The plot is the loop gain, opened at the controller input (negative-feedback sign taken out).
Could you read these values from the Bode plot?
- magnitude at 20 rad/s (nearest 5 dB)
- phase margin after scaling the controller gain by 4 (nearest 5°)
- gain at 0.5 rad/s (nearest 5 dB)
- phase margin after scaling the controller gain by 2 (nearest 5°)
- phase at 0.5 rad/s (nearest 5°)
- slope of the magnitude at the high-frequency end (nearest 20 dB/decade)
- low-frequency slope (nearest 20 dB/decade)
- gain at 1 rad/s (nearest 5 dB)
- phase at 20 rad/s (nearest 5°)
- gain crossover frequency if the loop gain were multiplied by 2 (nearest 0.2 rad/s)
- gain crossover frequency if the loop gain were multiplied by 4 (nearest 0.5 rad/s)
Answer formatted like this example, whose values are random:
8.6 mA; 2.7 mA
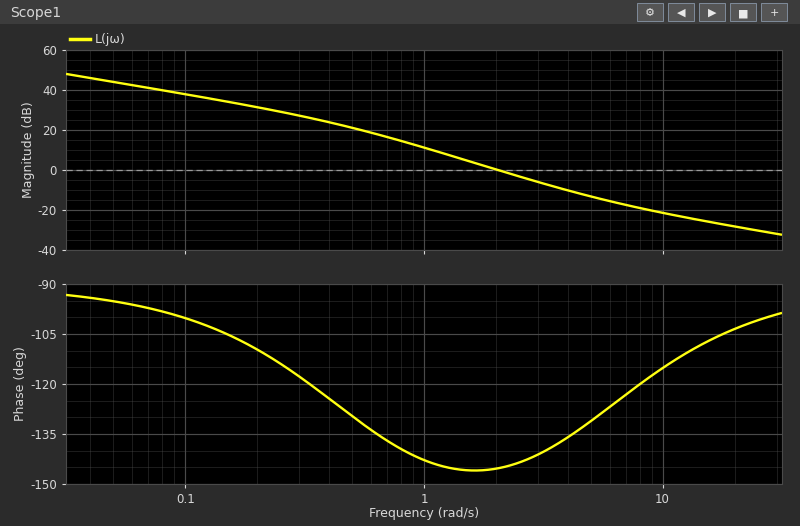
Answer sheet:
-30 dB; 45°; 20 dB; 40°; -130°; -20 dB/decade; -20 dB/decade; 10 dB; -105°; 3.0 rad/s; 4.5 rad/s
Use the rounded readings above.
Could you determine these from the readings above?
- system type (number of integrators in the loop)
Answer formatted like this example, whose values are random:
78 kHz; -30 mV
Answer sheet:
1
